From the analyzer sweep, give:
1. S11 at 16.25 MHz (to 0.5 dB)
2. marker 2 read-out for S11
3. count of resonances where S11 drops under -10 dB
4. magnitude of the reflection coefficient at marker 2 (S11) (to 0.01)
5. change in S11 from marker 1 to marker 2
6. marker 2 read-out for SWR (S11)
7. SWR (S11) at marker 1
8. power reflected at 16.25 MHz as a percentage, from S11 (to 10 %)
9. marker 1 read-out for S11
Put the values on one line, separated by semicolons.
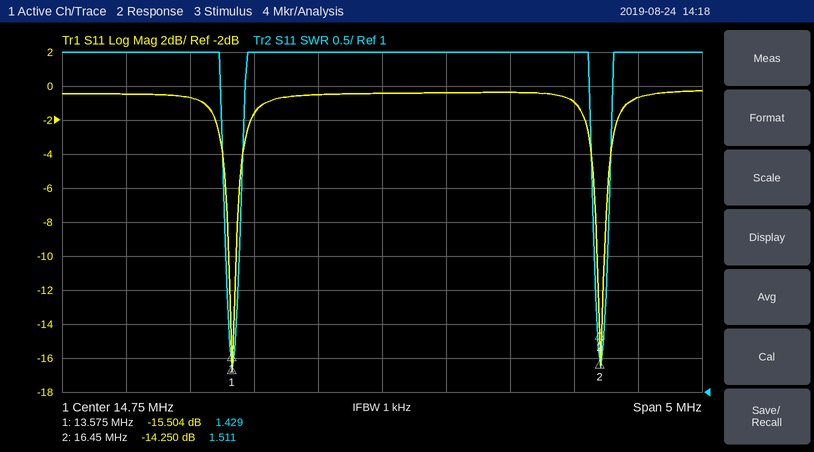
-1.0 dB; -14.250 dB; 2; 0.19; 1.254 dB; 1.511; 1.429; 80 %; -15.504 dB
